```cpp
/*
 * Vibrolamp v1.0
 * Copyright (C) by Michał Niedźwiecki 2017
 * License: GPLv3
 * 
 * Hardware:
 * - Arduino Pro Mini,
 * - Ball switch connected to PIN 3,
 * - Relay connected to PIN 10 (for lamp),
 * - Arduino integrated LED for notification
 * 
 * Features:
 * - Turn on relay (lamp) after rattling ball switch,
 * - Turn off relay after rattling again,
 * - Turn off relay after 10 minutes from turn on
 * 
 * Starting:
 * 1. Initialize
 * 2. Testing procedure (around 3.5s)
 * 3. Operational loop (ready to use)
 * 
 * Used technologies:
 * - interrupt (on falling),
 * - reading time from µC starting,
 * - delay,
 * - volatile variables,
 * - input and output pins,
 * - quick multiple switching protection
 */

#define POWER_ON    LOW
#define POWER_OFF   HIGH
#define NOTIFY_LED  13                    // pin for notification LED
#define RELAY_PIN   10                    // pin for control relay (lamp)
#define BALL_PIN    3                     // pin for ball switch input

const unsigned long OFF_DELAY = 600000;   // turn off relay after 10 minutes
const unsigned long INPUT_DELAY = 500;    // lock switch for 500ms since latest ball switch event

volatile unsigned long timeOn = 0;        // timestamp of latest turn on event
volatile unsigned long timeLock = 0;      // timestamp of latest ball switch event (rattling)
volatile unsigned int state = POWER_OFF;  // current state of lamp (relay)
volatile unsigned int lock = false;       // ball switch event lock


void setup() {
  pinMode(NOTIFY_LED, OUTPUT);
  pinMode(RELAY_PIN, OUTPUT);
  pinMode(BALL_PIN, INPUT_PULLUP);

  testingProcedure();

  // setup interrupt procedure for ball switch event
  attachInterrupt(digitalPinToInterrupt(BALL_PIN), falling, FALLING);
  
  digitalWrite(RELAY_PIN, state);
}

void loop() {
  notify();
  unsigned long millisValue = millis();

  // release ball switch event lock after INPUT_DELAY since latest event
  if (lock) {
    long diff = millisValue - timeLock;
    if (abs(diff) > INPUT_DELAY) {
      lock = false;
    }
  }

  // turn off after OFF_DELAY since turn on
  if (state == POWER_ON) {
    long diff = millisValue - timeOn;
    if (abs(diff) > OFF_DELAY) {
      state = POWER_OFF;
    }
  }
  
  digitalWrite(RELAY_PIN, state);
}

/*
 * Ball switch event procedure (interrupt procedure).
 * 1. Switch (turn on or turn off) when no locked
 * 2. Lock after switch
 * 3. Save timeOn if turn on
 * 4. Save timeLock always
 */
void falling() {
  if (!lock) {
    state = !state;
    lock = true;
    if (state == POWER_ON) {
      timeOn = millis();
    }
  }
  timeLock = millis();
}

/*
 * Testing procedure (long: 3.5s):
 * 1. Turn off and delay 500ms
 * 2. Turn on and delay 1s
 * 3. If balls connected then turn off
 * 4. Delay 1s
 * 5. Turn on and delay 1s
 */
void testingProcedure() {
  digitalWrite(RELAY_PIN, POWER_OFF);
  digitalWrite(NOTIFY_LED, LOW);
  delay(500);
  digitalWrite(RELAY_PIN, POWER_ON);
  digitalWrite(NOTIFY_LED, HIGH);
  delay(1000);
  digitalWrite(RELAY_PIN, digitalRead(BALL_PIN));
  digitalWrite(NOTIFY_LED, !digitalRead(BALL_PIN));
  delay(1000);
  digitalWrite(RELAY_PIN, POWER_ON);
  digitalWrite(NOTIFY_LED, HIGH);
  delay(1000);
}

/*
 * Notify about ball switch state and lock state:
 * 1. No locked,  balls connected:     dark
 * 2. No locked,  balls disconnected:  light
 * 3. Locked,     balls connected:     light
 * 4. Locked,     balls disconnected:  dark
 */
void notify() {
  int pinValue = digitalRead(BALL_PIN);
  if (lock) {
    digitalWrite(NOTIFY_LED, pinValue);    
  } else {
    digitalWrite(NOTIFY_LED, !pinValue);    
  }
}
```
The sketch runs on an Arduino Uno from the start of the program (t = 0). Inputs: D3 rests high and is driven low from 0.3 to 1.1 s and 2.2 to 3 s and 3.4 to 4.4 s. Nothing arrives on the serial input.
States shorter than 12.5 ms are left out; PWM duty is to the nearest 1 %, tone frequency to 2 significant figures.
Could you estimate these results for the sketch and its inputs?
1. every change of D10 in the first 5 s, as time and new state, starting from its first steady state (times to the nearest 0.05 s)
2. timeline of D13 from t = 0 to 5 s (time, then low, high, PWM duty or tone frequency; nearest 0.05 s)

0 s high; 0.5 s low; 1.5 s high; 2.5 s low; 3.5 s high
0 s low; 0.5 s high; 1.5 s low; 2.5 s high; 4.4 s low
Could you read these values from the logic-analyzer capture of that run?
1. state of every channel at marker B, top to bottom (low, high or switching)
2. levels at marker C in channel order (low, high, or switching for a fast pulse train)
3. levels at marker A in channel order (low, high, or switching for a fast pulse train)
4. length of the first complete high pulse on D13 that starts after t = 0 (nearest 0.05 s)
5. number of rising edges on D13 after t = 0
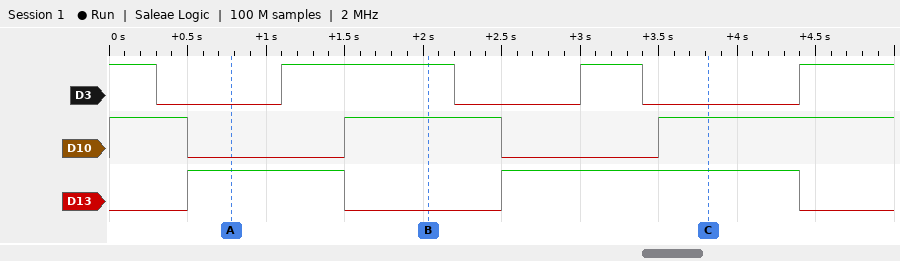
D3 high, D10 high, D13 low
D3 low, D10 high, D13 high
D3 low, D10 low, D13 high
1.00 s
2
